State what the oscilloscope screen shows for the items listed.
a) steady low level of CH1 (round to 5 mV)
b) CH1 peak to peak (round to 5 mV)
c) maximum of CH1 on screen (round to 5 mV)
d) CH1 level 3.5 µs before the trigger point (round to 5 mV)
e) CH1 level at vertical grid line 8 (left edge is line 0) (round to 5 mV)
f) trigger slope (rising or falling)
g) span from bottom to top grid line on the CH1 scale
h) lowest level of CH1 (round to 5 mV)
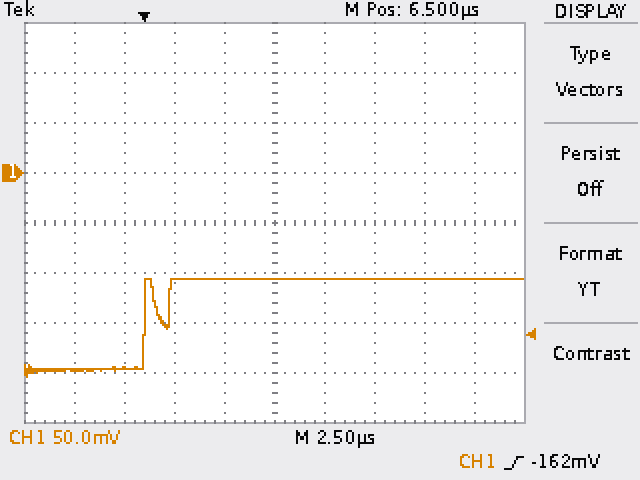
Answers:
-195 mV
100 mV
-105 mV
-195 mV
-105 mV
rising
400 mV
-205 mV
